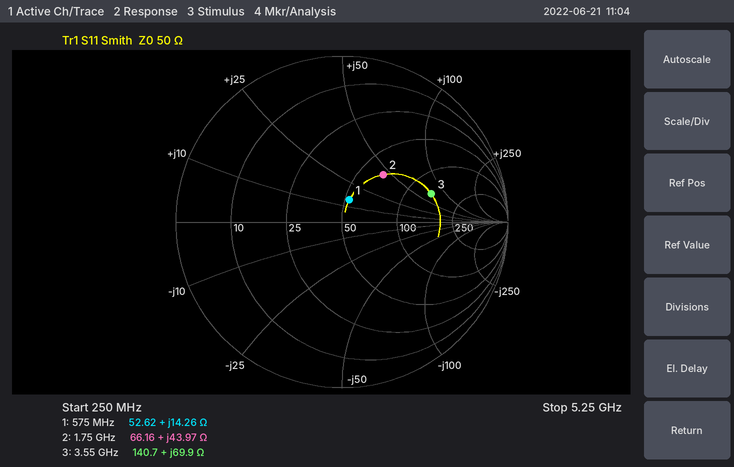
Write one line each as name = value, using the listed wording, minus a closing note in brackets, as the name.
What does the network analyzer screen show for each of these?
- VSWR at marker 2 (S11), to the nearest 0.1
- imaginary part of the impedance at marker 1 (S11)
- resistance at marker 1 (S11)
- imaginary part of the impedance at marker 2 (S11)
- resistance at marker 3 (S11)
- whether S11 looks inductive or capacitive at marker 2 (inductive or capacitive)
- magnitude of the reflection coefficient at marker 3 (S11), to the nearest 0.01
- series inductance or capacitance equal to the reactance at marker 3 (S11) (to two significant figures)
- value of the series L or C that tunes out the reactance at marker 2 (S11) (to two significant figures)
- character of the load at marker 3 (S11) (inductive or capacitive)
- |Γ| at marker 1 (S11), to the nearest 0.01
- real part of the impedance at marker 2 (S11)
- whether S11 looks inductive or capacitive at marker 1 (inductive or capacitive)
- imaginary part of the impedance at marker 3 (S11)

VSWR at marker 2 (S11), to the nearest 0.1 = 2.2
imaginary part of the impedance at marker 1 = +14.26 Ω
resistance at marker 1 = 52.62 Ω
imaginary part of the impedance at marker 2 = +43.97 Ω
resistance at marker 3 = 140.7 Ω
whether S11 looks inductive or capacitive at marker 2 = inductive
magnitude of the reflection coefficient at marker 3 (S11), to the nearest 0.01 = 0.56
series inductance or capacitance equal to the reactance at marker 3 (S11) = 3.1 nH
value of the series L or C that tunes out the reactance at marker 2 (S11) = 2.1 pF
character of the load at marker 3 (S11) = inductive
|Γ| at marker 1 (S11), to the nearest 0.01 = 0.14
real part of the impedance at marker 2 = 66.16 Ω
whether S11 looks inductive or capacitive at marker 1 = inductive
imaginary part of the impedance at marker 3 = +69.9 Ω
